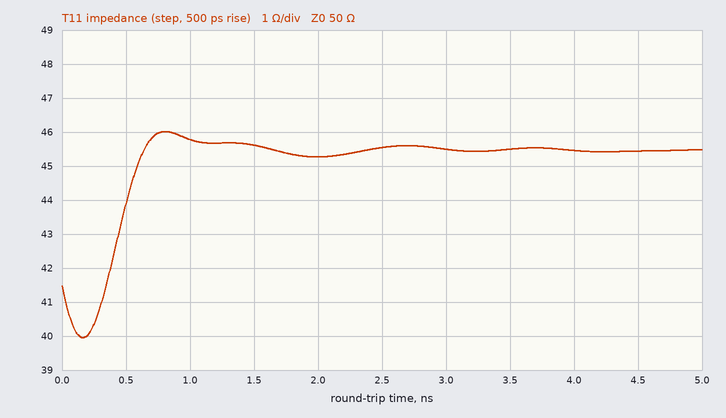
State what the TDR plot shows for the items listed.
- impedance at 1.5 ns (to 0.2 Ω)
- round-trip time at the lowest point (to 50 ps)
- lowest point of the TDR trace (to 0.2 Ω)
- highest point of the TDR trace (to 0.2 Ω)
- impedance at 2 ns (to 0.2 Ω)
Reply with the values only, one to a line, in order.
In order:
45.6 Ω
150 ps
40.0 Ω
46.0 Ω
45.2 Ω
